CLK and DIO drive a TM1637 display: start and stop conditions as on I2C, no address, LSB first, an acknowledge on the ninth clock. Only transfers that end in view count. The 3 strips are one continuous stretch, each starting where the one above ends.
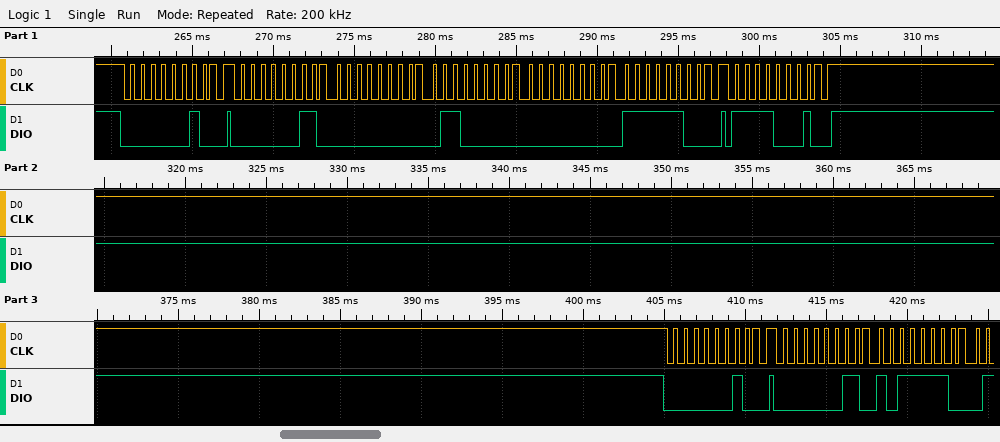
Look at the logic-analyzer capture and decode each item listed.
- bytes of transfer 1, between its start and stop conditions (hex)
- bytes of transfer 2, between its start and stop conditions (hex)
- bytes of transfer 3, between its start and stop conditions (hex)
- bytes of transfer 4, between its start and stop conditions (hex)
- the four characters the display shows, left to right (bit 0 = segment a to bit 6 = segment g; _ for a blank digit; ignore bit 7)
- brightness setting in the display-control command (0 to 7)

40
C0 00 06 00 3F
8F
40
_1_0
7
